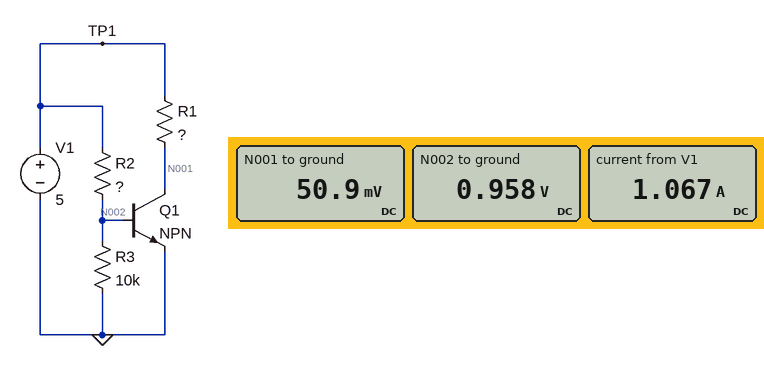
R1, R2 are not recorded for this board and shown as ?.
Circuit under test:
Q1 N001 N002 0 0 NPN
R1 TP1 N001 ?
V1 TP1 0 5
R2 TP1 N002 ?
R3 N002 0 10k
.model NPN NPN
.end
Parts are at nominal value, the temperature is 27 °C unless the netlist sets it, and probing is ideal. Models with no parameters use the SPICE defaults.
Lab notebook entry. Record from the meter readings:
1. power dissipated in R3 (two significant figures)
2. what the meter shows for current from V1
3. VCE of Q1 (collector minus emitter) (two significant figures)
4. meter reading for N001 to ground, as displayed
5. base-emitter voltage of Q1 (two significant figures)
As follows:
92 µW
1.067 A
51 mV
50.9 mV
960 mV
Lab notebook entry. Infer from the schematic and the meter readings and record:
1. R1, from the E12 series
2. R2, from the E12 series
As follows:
5.6 Ω
22 Ω
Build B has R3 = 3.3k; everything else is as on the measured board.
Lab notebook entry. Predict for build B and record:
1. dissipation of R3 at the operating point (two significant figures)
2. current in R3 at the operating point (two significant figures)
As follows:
280 µW
290 µA
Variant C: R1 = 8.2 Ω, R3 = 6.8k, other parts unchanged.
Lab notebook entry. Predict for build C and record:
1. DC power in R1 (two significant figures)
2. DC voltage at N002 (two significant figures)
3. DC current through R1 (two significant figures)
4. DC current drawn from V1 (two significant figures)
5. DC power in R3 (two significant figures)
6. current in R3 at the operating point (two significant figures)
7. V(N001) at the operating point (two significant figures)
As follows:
3.0 W
950 mV
600 mA
790 mA
130 µW
140 µA
44 mV
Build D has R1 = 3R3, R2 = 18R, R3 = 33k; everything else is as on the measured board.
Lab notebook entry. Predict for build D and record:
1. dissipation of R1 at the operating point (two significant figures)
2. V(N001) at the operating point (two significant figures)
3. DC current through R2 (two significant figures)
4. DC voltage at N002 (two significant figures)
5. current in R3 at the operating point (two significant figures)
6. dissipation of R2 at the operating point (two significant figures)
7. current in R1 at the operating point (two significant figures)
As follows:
7.4 W
58 mV
220 mA
970 mV
29 µA
900 mW
1.5 A
